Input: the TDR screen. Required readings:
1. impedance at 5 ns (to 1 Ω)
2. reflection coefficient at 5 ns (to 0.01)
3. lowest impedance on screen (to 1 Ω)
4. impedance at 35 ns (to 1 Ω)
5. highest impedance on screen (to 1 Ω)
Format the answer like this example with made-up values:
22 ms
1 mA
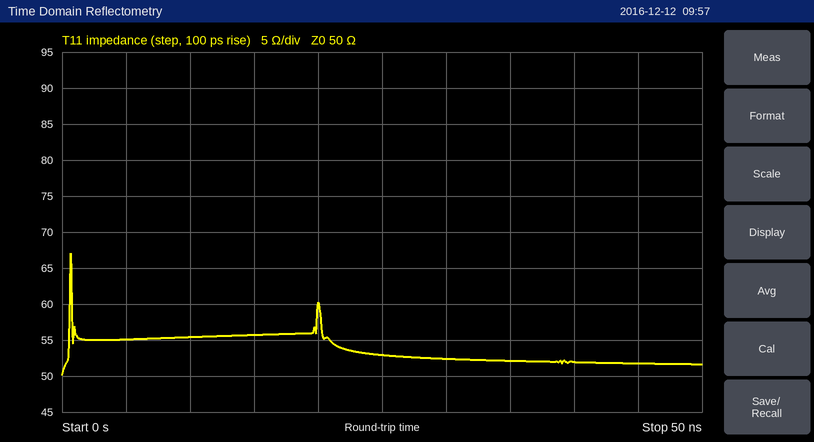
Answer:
55 Ω
+0.05
50 Ω
52 Ω
67 Ω
